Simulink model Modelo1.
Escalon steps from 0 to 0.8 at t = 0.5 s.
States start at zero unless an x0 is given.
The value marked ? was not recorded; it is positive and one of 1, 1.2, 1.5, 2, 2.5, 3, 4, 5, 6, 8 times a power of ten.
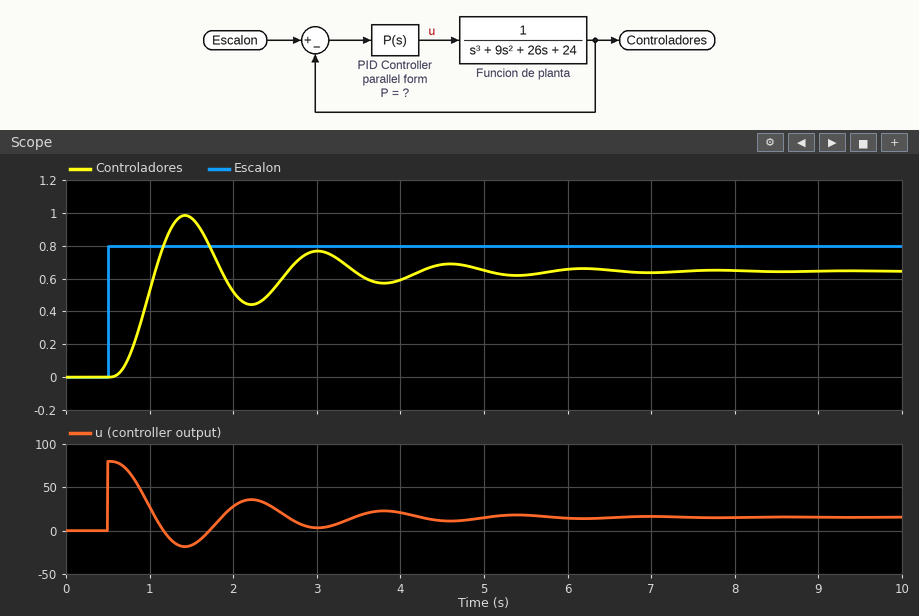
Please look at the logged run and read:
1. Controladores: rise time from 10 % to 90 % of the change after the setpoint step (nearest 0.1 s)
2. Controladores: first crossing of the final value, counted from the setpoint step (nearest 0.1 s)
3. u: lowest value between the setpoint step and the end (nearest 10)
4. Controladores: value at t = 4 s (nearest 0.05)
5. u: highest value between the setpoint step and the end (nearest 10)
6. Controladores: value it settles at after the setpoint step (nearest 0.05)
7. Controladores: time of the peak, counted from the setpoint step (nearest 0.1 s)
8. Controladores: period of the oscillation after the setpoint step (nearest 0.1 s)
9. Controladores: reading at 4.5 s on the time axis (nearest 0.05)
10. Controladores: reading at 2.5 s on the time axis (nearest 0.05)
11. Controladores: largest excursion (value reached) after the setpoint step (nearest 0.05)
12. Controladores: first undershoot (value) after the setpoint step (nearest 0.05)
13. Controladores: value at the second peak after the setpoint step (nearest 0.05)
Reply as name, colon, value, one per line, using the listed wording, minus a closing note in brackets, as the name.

Controladores: rise time from 10 % to 90 % of the change after the setpoint step: 0.3 s
Controladores: first crossing of the final value, counted from the setpoint step: 0.6 s
u: lowest value between the setpoint step and the end: -20
Controladores: value at t = 4 s: 0.60
u: highest value between the setpoint step and the end: 80
Controladores: value it settles at after the setpoint step: 0.65
Controladores: time of the peak, counted from the setpoint step: 0.9 s
Controladores: period of the oscillation after the setpoint step: 1.6 s
Controladores: reading at 4.5 s on the time axis: 0.70
Controladores: reading at 2.5 s on the time axis: 0.55
Controladores: largest excursion (value reached) after the setpoint step: 1.00
Controladores: first undershoot (value) after the setpoint step: 0.45
Controladores: value at the second peak after the setpoint step: 0.75
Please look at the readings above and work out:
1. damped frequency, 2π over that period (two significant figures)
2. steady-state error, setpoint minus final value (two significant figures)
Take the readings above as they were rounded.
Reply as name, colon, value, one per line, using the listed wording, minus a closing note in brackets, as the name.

damped frequency, 2π over that period: 3.9 rad/s
steady-state error, setpoint minus final value: 0.15
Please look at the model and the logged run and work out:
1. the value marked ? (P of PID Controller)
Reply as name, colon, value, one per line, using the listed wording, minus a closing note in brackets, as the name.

the value marked ?: 100
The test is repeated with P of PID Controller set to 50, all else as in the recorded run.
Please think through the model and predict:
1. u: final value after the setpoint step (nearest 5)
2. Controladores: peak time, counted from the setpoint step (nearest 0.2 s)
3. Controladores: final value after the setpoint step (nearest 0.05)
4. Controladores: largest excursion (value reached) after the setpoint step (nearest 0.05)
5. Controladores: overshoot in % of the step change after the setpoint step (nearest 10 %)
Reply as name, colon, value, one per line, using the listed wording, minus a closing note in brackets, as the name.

u: final value after the setpoint step: 15
Controladores: peak time, counted from the setpoint step: 1.2 s
Controladores: final value after the setpoint step: 0.55
Controladores: largest excursion (value reached) after the setpoint step: 0.70
Controladores: overshoot in % of the step change after the setpoint step: 30 %
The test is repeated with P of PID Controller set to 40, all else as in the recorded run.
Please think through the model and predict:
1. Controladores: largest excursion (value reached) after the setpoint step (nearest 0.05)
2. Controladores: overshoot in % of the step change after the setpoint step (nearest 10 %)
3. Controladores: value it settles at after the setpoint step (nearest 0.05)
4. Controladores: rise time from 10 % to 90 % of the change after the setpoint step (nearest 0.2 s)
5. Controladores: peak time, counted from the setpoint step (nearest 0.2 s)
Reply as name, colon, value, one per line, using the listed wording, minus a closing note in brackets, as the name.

Controladores: largest excursion (value reached) after the setpoint step: 0.60
Controladores: overshoot in % of the step change after the setpoint step: 20 %
Controladores: value it settles at after the setpoint step: 0.50
Controladores: rise time from 10 % to 90 % of the change after the setpoint step: 0.6 s
Controladores: peak time, counted from the setpoint step: 1.2 s
